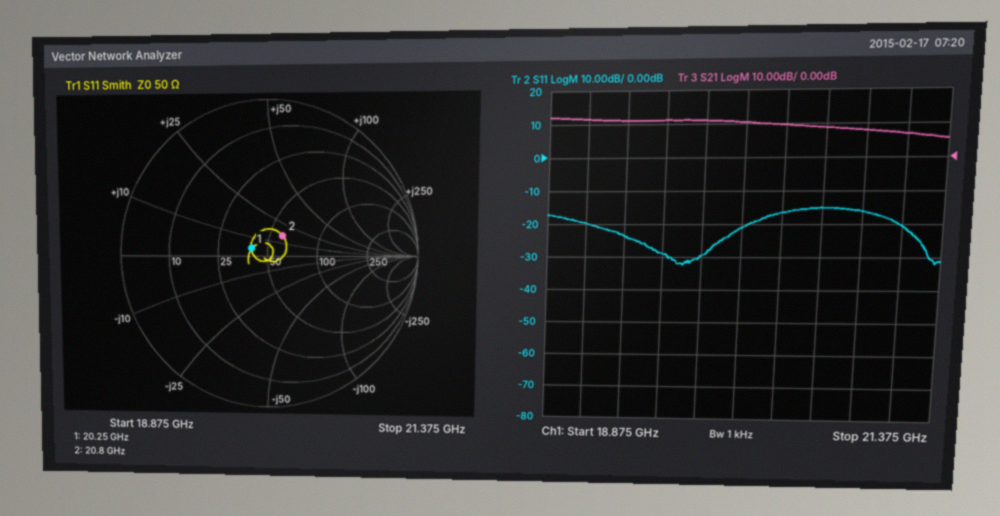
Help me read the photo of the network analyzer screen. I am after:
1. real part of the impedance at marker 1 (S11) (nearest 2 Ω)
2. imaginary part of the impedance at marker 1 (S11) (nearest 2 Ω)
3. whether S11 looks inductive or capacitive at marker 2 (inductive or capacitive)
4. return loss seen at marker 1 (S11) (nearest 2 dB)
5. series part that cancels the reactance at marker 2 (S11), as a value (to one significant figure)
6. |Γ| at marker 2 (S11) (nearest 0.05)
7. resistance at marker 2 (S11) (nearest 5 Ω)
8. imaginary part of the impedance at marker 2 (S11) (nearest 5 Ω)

40 Ω
+4 Ω
inductive
18 dB
500 fF
0.15
60 Ω
+15 Ω
